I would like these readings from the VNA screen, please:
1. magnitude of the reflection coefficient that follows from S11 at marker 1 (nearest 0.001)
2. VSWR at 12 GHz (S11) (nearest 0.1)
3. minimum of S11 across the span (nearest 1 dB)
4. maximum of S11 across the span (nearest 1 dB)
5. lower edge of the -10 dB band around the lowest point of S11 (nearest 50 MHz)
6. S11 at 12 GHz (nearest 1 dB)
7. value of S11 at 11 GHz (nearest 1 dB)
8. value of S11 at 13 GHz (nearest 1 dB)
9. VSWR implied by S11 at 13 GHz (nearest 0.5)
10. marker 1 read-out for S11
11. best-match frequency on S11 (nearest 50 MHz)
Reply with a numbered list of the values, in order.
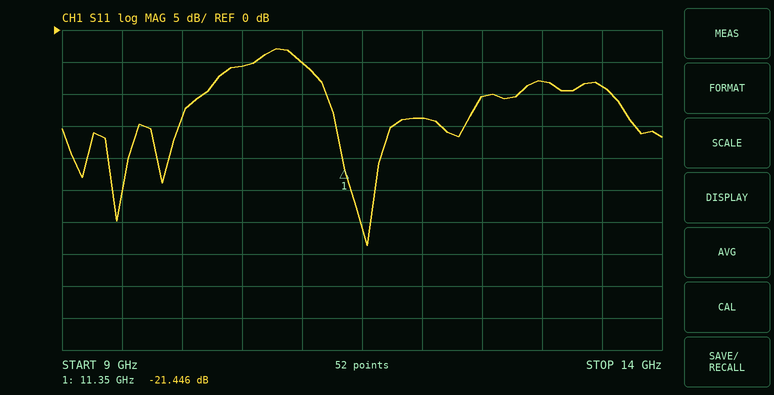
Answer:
1. 0.085
2. 1.5
3. -34 dB
4. -3 dB
5. 11.20 GHz
6. -14 dB
7. -5 dB
8. -8 dB
9. 2.5
10. -21.446 dB
11. 11.55 GHz
